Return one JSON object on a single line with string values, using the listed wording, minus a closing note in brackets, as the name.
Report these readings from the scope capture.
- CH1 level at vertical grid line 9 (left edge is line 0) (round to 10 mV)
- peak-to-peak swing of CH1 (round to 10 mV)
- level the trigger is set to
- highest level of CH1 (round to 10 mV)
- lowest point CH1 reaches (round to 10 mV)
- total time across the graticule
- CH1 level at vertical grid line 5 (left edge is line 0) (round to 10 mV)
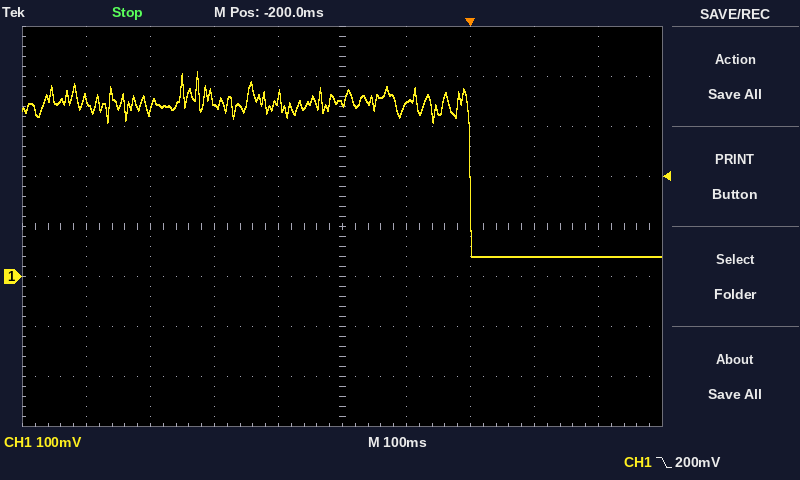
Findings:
{"CH1 level at vertical grid line 9 (left edge is line 0)": "40 mV", "peak-to-peak swing of CH1": "370 mV", "level the trigger is set to": "200 mV", "highest level of CH1": "410 mV", "lowest point CH1 reaches": "40 mV", "total time across the graticule": "1 s", "CH1 level at vertical grid line 5 (left edge is line 0)": "350 mV"}
